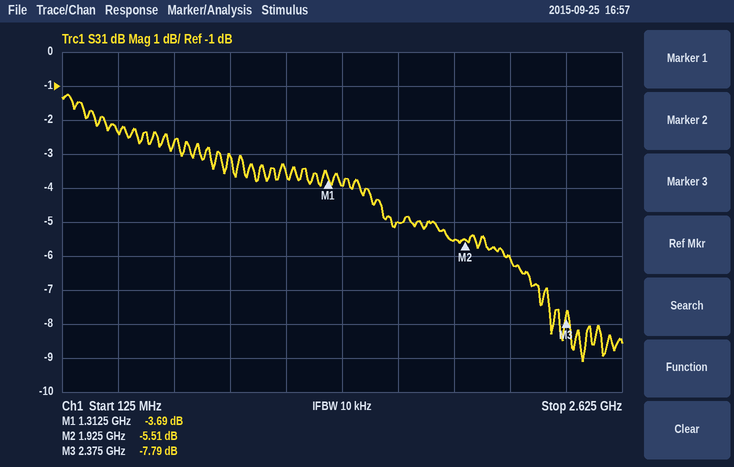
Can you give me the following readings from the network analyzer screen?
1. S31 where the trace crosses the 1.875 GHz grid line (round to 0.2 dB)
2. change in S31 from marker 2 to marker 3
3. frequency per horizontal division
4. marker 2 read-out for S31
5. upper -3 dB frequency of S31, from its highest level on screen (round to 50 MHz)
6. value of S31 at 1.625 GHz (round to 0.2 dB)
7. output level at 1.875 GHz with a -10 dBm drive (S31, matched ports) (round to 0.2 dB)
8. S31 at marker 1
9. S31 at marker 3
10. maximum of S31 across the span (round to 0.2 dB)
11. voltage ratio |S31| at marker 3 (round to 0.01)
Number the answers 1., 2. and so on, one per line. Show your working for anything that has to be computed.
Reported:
1. -5.6 dB
2. -7.79 − (-5.51) = -2.28 dB
3. 250 MHz
4. -5.51 dB
5. 1.50 GHz
6. -5.0 dB
7. -10 dBm + (-5.6 dB) = -15.6 dBm
8. -3.69 dB
9. -7.79 dB
10. -1.2 dB
11. 10^(-7.79/20) ≈ 0.41
